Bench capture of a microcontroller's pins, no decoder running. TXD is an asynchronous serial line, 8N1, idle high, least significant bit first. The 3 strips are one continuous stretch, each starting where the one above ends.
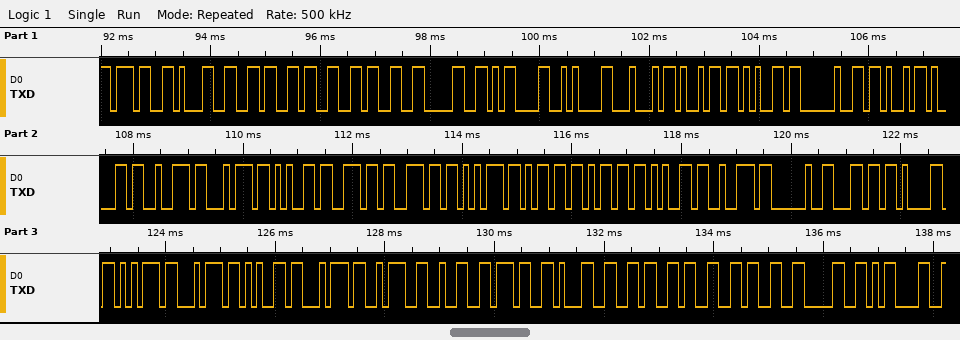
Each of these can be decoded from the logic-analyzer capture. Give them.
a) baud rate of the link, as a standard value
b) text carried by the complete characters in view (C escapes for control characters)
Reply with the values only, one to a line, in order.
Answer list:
9600 baud
"716330\r\nDie Kartennummer lautet:2716330\r"
